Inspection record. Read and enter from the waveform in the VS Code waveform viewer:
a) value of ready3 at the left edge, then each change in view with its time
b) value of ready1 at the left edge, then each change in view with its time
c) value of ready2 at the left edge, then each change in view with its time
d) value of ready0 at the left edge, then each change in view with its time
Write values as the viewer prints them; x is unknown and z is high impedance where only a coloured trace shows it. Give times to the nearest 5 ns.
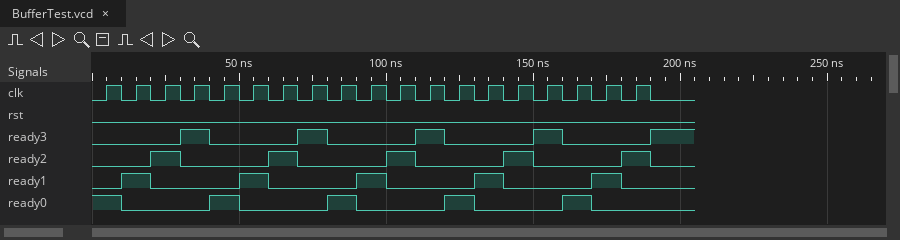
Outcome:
0, 1 at 30 ns, 0 at 40 ns, 1 at 70 ns, 0 at 80 ns, 1 at 110 ns, 0 at 120 ns, 1 at 150 ns, 0 at 160 ns, 1 at 190 ns
0, 1 at 10 ns, 0 at 20 ns, 1 at 50 ns, 0 at 60 ns, 1 at 90 ns, 0 at 100 ns, 1 at 130 ns, 0 at 140 ns, 1 at 170 ns, 0 at 180 ns
0, 1 at 20 ns, 0 at 30 ns, 1 at 60 ns, 0 at 70 ns, 1 at 100 ns, 0 at 110 ns, 1 at 140 ns, 0 at 150 ns, 1 at 180 ns, 0 at 190 ns
1, 0 at 10 ns, 1 at 40 ns, 0 at 50 ns, 1 at 80 ns, 0 at 90 ns, 1 at 120 ns, 0 at 130 ns, 1 at 160 ns, 0 at 170 ns
